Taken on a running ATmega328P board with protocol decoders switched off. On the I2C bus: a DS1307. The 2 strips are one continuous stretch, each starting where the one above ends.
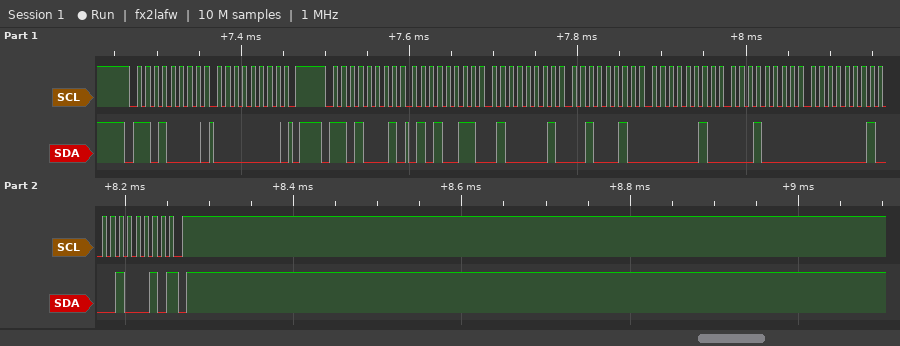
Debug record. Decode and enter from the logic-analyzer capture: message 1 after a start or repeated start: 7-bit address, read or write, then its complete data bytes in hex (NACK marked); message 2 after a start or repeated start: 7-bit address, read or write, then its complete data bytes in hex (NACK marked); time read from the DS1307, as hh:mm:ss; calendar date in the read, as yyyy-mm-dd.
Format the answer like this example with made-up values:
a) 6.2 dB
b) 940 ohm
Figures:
a) 0x68 write: 00
b) 0x68 read: 53 41 22 02 10 01 22 NACK
c) 22:41:53
d) 2022-01-10
